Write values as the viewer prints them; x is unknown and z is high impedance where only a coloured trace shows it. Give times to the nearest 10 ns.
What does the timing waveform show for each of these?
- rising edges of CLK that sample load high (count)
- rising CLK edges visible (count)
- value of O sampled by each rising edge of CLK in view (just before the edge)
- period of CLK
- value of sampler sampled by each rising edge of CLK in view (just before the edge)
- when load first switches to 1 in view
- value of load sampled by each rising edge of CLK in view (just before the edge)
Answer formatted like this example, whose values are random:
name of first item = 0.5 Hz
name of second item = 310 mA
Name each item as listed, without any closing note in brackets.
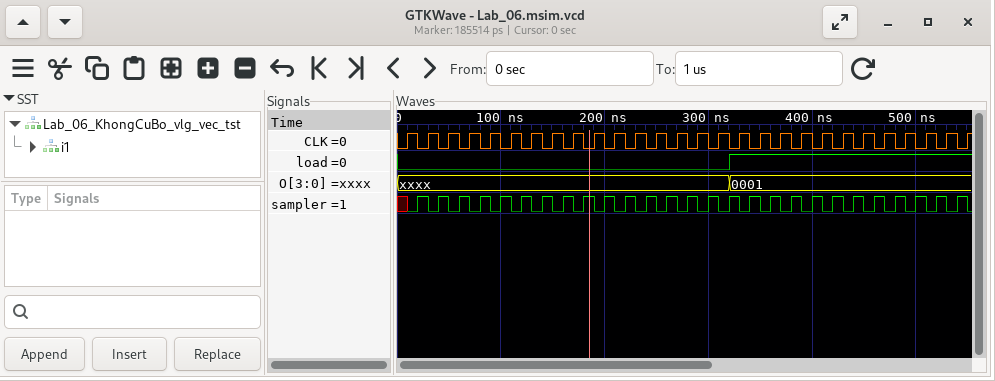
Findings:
rising edges of CLK that sample load high = 12
rising CLK edges visible = 28
value of O sampled by each rising edge of CLK in view = xxxx, xxxx, xxxx, xxxx, xxxx, xxxx, xxxx, xxxx, xxxx, xxxx, xxxx, xxxx, xxxx, xxxx, xxxx, xxxx, 0001, 0001, 0001, 0001, 0001, 0001, 0001, 0001, 0001, 0001, 0001, 0001
period of CLK = 20 ns
value of sampler sampled by each rising edge of CLK in view = x 1 1 1 1 1 1 1 1 1 1 1 1 1 1 1 1 1 1 1 1 1 1 1 1 1 1 1
when load first switches to 1 in view = 320 ns
value of load sampled by each rising edge of CLK in view = 0 0 0 0 0 0 0 0 0 0 0 0 0 0 0 0 1 1 1 1 1 1 1 1 1 1 1 1
